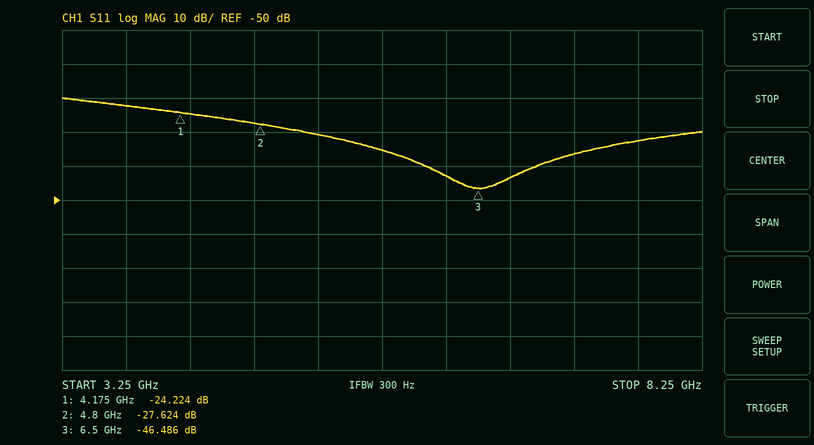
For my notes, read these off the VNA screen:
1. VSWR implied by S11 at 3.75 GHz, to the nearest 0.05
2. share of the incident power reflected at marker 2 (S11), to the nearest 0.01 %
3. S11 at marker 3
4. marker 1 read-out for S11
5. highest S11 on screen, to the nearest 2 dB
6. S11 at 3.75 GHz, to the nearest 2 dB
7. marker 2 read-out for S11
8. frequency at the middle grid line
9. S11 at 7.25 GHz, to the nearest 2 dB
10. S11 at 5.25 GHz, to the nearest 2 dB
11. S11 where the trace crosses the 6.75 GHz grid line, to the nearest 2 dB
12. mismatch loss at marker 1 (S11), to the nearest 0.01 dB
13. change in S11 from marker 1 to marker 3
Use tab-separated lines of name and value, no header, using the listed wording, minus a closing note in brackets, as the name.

VSWR implied by S11 at 3.75 GHz, to the nearest 0.05	1.15
share of the incident power reflected at marker 2 (S11), to the nearest 0.01 %	0.17 %
S11 at marker 3	-46.486 dB
marker 1 read-out for S11	-24.224 dB
highest S11 on screen, to the nearest 2 dB	-20 dB
S11 at 3.75 GHz, to the nearest 2 dB	-22 dB
marker 2 read-out for S11	-27.624 dB
frequency at the middle grid line	5.75 GHz
S11 at 7.25 GHz, to the nearest 2 dB	-36 dB
S11 at 5.25 GHz, to the nearest 2 dB	-30 dB
S11 where the trace crosses the 6.75 GHz grid line, to the nearest 2 dB	-44 dB
mismatch loss at marker 1 (S11), to the nearest 0.01 dB	0.02 dB
change in S11 from marker 1 to marker 3	-22.262 dB
